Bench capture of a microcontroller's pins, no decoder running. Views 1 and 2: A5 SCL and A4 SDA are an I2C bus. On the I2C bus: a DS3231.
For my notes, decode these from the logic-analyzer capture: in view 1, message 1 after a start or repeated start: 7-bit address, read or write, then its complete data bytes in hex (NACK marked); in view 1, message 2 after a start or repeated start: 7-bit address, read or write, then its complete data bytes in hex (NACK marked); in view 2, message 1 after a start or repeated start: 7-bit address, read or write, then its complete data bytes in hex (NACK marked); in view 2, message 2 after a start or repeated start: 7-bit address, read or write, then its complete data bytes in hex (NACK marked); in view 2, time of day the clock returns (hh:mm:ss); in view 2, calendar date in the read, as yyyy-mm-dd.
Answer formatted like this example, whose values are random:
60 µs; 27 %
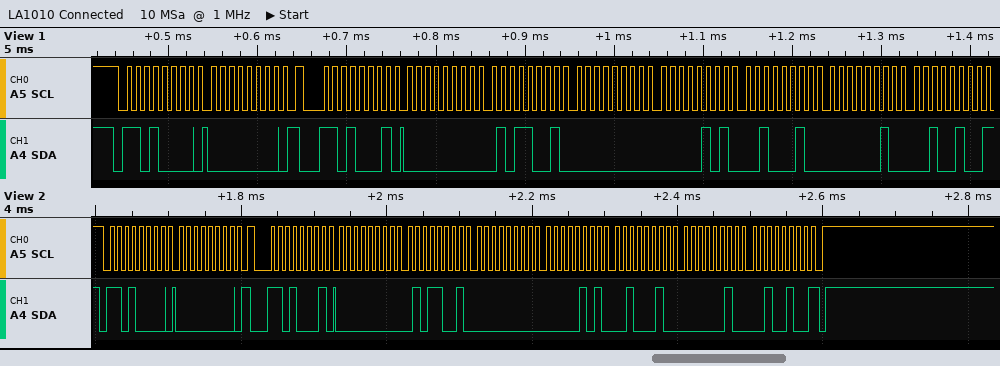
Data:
0x68 write: 00; 0x68 read: 00 59 00 05 22 02 24 NACK; 0x68 write: 00; 0x68 read: 00 59 00 05 22 02 24 NACK; 00:59:00; 2024-02-22
